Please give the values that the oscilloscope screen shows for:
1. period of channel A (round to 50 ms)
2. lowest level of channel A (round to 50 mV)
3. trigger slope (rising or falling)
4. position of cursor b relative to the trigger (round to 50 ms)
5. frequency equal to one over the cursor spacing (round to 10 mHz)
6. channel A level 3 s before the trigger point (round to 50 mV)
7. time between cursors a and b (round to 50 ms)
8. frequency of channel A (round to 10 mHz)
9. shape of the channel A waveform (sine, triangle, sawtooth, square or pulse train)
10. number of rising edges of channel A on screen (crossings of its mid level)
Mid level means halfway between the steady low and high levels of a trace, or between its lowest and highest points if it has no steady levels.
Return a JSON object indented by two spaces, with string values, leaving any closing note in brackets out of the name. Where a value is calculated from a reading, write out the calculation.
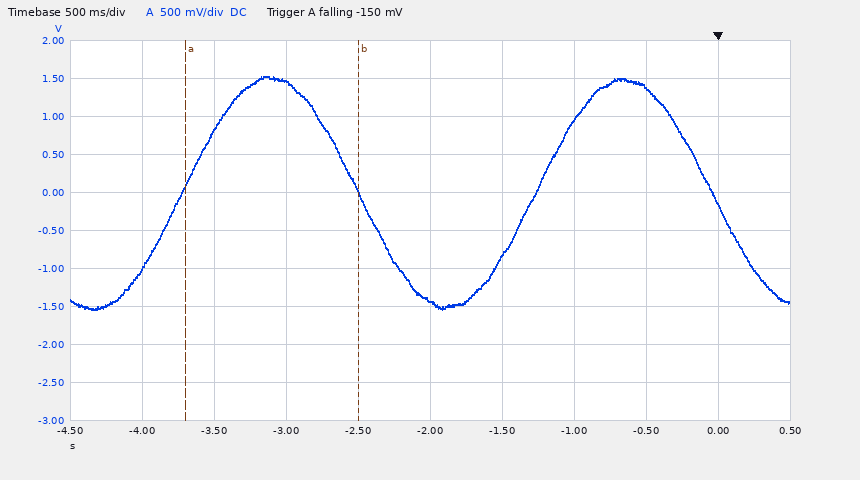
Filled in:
{
  "period of channel A": "2.45 s",
  "lowest level of channel A": "-1.55 V",
  "trigger slope": "falling",
  "position of cursor b relative to the trigger": "-2.50 s",
  "frequency equal to one over the cursor spacing": "1 / 1.20 s ≈ 830 mHz",
  "channel A level 3 s before the trigger point": "1.45 V",
  "time between cursors a and b": "1.20 s",
  "frequency of channel A": "1 / 2.45 s ≈ 408 mHz, so 410 mHz to the nearest 10 mHz",
  "shape of the channel A waveform": "sine",
  "number of rising edges of channel A on screen": "2"
}
